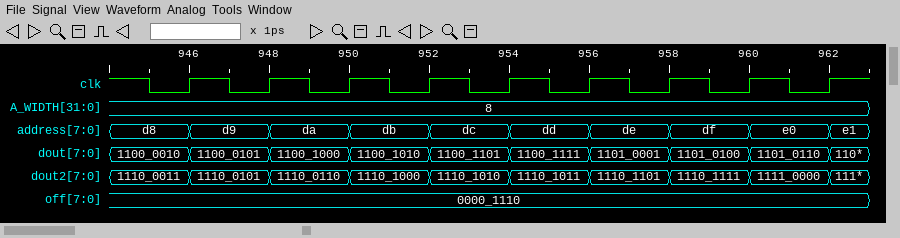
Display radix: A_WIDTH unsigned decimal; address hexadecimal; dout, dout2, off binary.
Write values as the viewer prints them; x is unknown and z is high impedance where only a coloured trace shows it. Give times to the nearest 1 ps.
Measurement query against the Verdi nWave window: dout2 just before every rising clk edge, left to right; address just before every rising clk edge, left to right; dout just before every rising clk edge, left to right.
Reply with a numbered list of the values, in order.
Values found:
1. 1110_0011, 1110_0101, 1110_0110, 1110_1000, 1110_1010, 1110_1011, 1110_1101, 1110_1111, 1111_0000
2. d8, d9, da, db, dc, dd, de, df, e0
3. 1100_0010, 1100_0101, 1100_1000, 1100_1010, 1100_1101, 1100_1111, 1101_0001, 1101_0100, 1101_0110
